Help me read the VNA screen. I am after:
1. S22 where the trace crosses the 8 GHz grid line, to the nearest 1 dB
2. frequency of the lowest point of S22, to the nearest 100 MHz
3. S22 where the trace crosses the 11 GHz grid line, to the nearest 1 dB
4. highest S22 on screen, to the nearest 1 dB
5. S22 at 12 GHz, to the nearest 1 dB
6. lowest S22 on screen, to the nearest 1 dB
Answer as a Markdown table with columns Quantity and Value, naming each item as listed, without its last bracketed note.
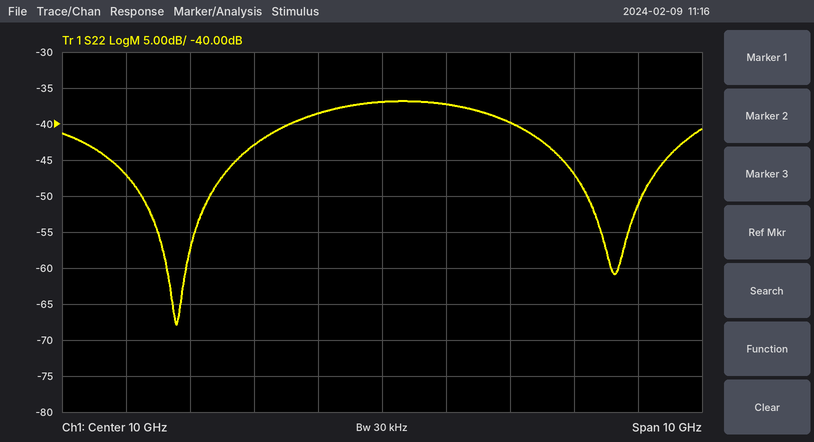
| Quantity | Value |
|---|---|
| S22 where the trace crosses the 8 GHz grid line, to the nearest 1 dB | -43 dB |
| frequency of the lowest point of S22, to the nearest 100 MHz | 6.8 GHz |
| S22 where the trace crosses the 11 GHz grid line, to the nearest 1 dB | -37 dB |
| highest S22 on screen, to the nearest 1 dB | -37 dB |
| S22 at 12 GHz, to the nearest 1 dB | -40 dB |
| lowest S22 on screen, to the nearest 1 dB | -68 dB |
